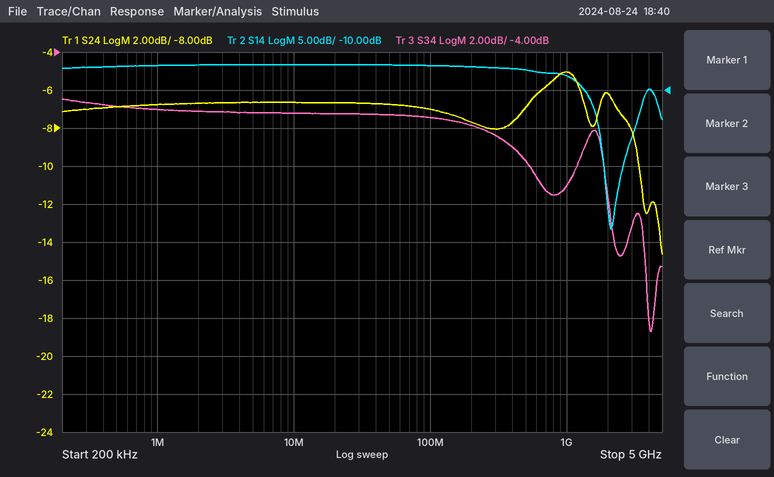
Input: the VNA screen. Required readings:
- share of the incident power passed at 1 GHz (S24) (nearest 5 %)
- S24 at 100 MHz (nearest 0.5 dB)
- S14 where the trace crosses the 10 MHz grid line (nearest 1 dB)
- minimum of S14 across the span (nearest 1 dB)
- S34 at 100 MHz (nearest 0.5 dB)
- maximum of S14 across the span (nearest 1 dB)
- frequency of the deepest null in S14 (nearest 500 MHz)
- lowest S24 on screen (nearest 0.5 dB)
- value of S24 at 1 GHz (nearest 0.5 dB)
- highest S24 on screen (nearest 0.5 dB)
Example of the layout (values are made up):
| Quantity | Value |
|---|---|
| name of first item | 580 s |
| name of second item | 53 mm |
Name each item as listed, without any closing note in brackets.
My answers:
| Quantity | Value |
|---|---|
| share of the incident power passed at 1 GHz (S24) | 30 % |
| S24 at 100 MHz | -7.0 dB |
| S14 where the trace crosses the 10 MHz grid line | -7 dB |
| minimum of S14 across the span | -28 dB |
| S34 at 100 MHz | -7.5 dB |
| maximum of S14 across the span | -7 dB |
| frequency of the deepest null in S14 | 2.0 GHz |
| lowest S24 on screen | -14.5 dB |
| value of S24 at 1 GHz | -5.0 dB |
| highest S24 on screen | -5.0 dB |
